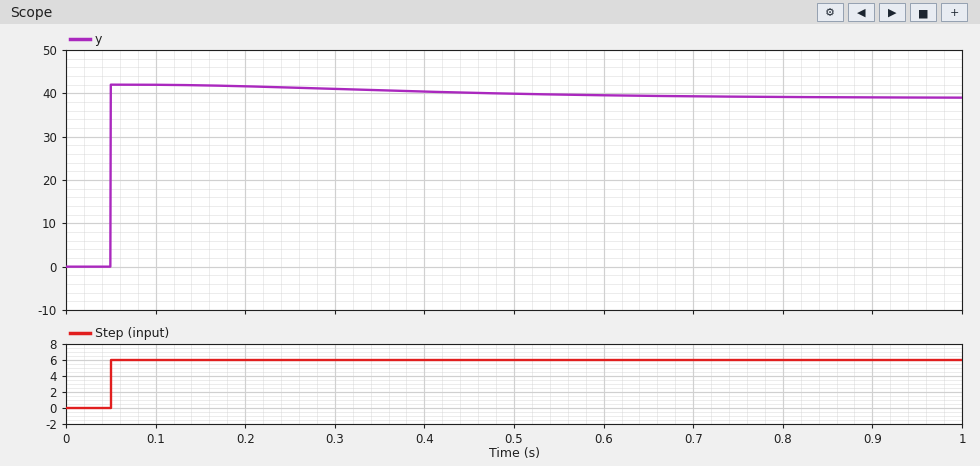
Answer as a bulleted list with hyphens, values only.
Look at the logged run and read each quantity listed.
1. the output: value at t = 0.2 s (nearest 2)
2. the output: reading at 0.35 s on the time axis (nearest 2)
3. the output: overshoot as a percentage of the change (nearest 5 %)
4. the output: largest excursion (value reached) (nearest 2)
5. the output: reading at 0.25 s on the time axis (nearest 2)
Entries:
- 42
- 40
- 10 %
- 42
- 42
